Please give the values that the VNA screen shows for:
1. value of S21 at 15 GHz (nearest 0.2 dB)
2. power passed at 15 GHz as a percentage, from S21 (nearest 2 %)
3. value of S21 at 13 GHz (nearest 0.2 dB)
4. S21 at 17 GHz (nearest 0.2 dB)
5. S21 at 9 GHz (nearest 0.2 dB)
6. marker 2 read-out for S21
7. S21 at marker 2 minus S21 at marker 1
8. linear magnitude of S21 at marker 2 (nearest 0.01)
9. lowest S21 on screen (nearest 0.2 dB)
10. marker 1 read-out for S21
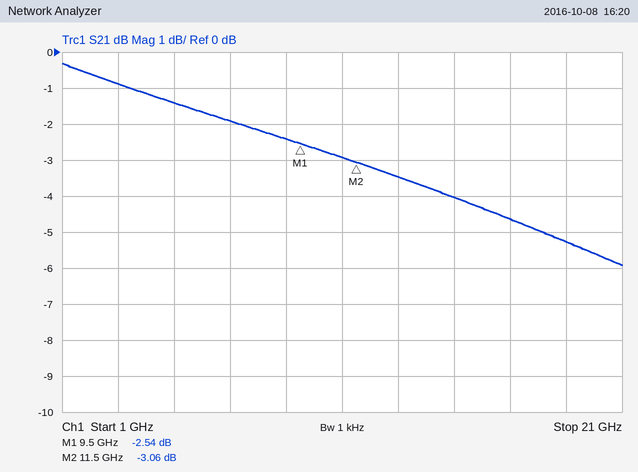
-4.0 dB
40 %
-3.4 dB
-4.6 dB
-2.4 dB
-3.06 dB
-0.52 dB
0.70
-6.0 dB
-2.54 dB
